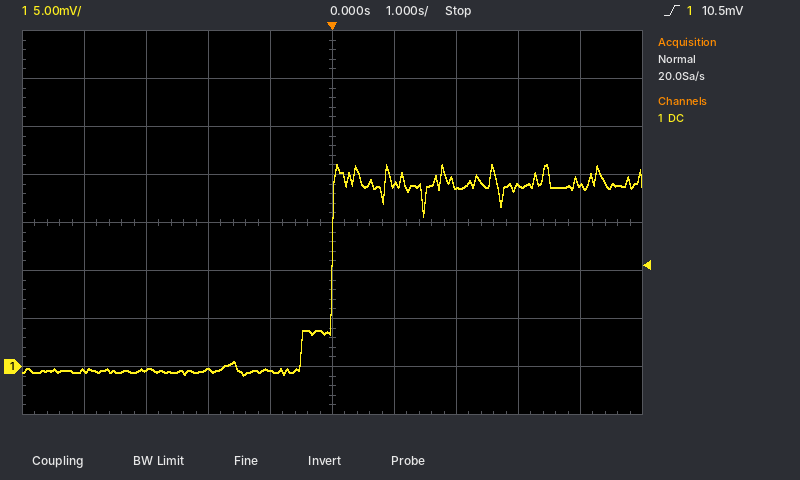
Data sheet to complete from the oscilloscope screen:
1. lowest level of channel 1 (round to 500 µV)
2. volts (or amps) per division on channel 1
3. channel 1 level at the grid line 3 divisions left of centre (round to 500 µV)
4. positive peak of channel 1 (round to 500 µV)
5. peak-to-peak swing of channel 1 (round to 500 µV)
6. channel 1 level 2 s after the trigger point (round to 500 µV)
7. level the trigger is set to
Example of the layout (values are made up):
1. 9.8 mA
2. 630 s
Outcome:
1. -1.0 mV
2. 5 mV
3. -500 µV
4. 21.0 mV
5. 22.0 mV
6. 19.0 mV
7. 10.5 mV
